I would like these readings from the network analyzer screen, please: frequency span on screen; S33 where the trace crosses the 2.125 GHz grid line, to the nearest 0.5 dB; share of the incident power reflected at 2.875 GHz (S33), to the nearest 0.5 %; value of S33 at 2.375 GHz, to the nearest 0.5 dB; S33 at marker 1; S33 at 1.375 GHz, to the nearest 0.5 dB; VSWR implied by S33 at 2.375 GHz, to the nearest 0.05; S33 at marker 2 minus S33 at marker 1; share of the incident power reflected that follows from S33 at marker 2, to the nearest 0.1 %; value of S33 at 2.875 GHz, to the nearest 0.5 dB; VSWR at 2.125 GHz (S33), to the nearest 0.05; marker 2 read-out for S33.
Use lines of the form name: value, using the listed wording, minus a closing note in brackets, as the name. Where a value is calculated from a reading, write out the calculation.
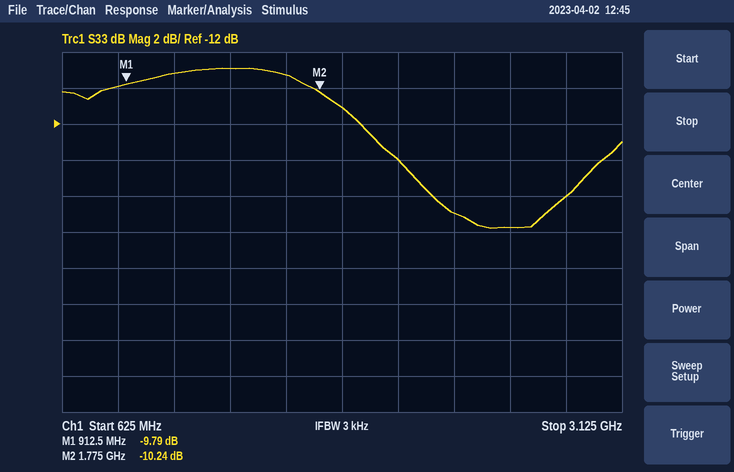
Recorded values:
frequency span on screen: 2.5 GHz
S33 where the trace crosses the 2.125 GHz grid line, to the nearest 0.5 dB: -14.0 dB
share of the incident power reflected at 2.875 GHz (S33), to the nearest 0.5 %: 10^(-16/10) ≈ 2.5 %
value of S33 at 2.375 GHz, to the nearest 0.5 dB: -17.0 dB
S33 at marker 1: -9.79 dB
S33 at 1.375 GHz, to the nearest 0.5 dB: -9.0 dB
VSWR implied by S33 at 2.375 GHz, to the nearest 0.05: |Γ| = 10^(-17/20) = 0.1413; VSWR = (1 + 0.1413)/(1 − 0.1413) ≈ 1.33, so 1.35 to the nearest 0.05
S33 at marker 2 minus S33 at marker 1: -10.24 − (-9.79) = -0.45 dB
share of the incident power reflected that follows from S33 at marker 2, to the nearest 0.1 %: 10^(-10.24/10) ≈ 9.5 %
value of S33 at 2.875 GHz, to the nearest 0.5 dB: -16.0 dB
VSWR at 2.125 GHz (S33), to the nearest 0.05: |Γ| = 10^(-14/20) = 0.1995; VSWR = (1 + 0.1995)/(1 − 0.1995) ≈ 1.50
marker 2 read-out for S33: -10.24 dB
